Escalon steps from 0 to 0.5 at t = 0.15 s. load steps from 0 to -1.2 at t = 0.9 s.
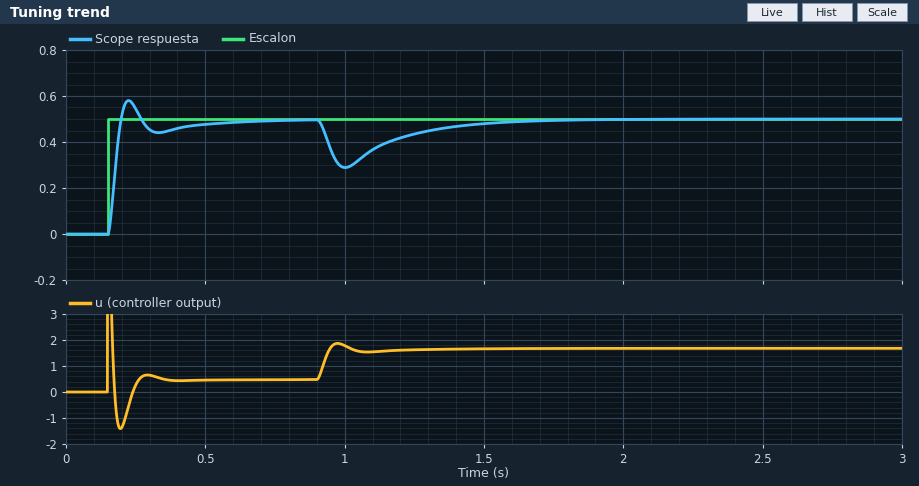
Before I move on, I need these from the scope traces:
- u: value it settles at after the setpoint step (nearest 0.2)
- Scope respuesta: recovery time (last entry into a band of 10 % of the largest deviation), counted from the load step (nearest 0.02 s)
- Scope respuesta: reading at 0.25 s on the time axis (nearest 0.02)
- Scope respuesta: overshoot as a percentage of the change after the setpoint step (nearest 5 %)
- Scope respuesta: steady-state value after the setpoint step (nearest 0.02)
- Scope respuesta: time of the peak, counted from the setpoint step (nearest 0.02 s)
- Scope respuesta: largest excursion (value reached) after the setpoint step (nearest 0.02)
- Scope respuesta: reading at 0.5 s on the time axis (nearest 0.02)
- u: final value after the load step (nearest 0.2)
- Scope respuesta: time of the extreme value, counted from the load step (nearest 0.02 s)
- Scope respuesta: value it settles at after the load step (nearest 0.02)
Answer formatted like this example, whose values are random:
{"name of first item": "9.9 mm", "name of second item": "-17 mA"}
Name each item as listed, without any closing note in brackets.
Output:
{"u: value it settles at after the setpoint step": "0.4", "Scope respuesta: recovery time (last entry into a band of 10 % of the largest deviation), counted from the load step": "0.60 s", "Scope respuesta: reading at 0.25 s on the time axis": "0.54", "Scope respuesta: overshoot as a percentage of the change after the setpoint step": "15 %", "Scope respuesta: steady-state value after the setpoint step": "0.50", "Scope respuesta: time of the peak, counted from the setpoint step": "0.08 s", "Scope respuesta: largest excursion (value reached) after the setpoint step": "0.58", "Scope respuesta: reading at 0.5 s on the time axis": "0.48", "u: final value after the load step": "1.6", "Scope respuesta: time of the extreme value, counted from the load step": "0.10 s", "Scope respuesta: value it settles at after the load step": "0.50"}
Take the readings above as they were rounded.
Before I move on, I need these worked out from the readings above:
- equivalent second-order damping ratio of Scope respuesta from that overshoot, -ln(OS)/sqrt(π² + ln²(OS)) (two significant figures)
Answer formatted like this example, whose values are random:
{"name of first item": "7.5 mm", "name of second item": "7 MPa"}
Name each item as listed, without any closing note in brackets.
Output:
{"equivalent second-order damping ratio of Scope respuesta from that overshoot, -ln(OS)/sqrt(π² + ln²(OS))": "0.52"}
